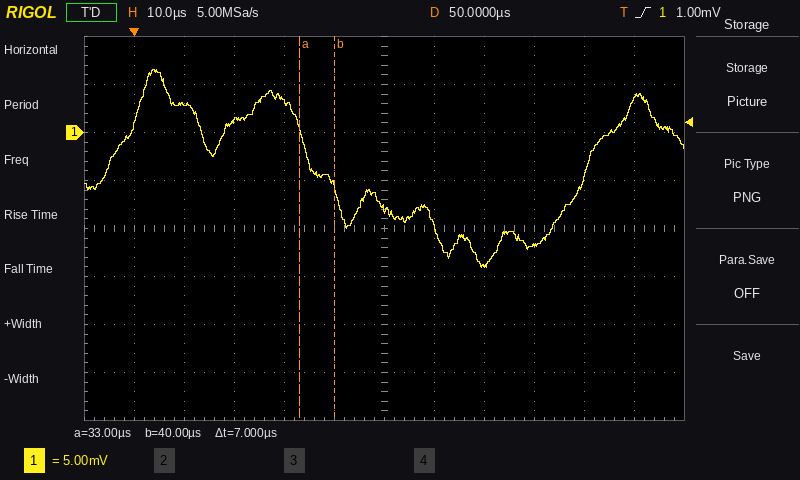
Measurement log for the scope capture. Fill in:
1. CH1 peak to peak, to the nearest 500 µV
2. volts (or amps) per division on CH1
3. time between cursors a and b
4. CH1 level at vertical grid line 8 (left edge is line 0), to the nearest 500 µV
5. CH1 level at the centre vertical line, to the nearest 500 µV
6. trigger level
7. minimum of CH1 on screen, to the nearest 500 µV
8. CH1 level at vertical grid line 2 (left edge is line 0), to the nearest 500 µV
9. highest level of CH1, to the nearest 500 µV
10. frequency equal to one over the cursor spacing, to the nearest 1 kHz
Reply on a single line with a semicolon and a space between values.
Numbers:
20.5 mV; 5 mV; 7 µs; -14.0 mV; -8.0 mV; 1.00 mV; -14.0 mV; 3.0 mV; 6.5 mV; 143 kHz
